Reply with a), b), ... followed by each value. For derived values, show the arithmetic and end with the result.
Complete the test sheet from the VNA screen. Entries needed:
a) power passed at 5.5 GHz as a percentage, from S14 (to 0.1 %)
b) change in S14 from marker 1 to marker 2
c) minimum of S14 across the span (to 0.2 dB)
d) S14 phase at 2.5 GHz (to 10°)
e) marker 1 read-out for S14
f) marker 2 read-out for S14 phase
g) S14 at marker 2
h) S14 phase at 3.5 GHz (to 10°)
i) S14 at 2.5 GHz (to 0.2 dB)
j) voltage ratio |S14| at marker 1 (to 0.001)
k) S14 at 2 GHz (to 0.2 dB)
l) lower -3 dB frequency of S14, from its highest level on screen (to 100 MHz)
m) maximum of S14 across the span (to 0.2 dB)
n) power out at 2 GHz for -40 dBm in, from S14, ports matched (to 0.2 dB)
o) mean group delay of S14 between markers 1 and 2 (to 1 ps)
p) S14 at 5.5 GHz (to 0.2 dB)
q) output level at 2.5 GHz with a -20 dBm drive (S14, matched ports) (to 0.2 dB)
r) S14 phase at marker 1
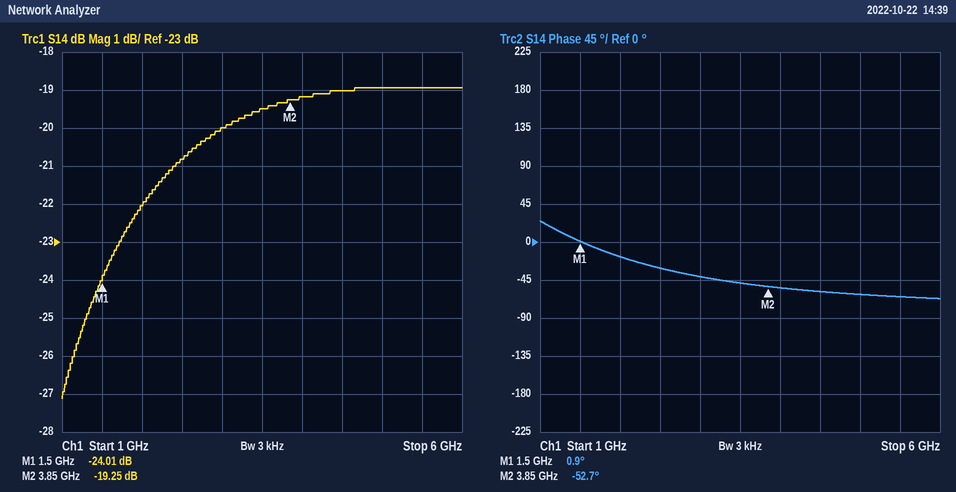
a) 10^(-19/10) ≈ 1.3 %
b) -19.25 − (-24.01) = 4.76 dB
c) -27.2 dB
d) -30°
e) -24.01 dB
f) -52.7°
g) -19.25 dB
h) -50°
i) -20.8 dB
j) 10^(-24.01/20) ≈ 0.063
k) -22.0 dB
l) 2.0 GHz
m) -19.0 dB
n) -40 dBm + (-22.0 dB) = -62.0 dBm
o) −(-52.7° − (0.9°))/(360° × 2.35 GHz) ≈ 63 ps
p) -19.0 dB
q) -20 dBm + (-20.8 dB) = -40.8 dBm
r) 0.9°
